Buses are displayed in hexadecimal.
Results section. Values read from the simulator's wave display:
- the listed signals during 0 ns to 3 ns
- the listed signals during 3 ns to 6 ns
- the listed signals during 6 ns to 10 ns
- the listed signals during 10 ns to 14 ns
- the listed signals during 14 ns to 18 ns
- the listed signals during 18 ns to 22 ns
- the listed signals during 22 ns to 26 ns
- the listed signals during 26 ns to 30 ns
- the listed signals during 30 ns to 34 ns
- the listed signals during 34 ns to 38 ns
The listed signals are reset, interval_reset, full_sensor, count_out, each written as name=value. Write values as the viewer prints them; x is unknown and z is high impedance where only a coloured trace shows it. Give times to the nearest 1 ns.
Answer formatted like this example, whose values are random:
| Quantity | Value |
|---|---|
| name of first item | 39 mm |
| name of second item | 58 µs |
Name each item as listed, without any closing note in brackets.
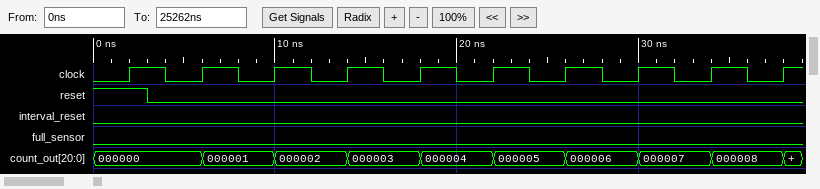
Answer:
| Quantity | Value |
|---|---|
| the listed signals during 0 ns to 3 ns | reset=1, interval_reset=0, full_sensor=0, count_out=000000 |
| the listed signals during 3 ns to 6 ns | reset=0, interval_reset=0, full_sensor=0, count_out=000000 |
| the listed signals during 6 ns to 10 ns | reset=0, interval_reset=0, full_sensor=0, count_out=000001 |
| the listed signals during 10 ns to 14 ns | reset=0, interval_reset=0, full_sensor=0, count_out=000002 |
| the listed signals during 14 ns to 18 ns | reset=0, interval_reset=0, full_sensor=0, count_out=000003 |
| the listed signals during 18 ns to 22 ns | reset=0, interval_reset=0, full_sensor=0, count_out=000004 |
| the listed signals during 22 ns to 26 ns | reset=0, interval_reset=0, full_sensor=0, count_out=000005 |
| the listed signals during 26 ns to 30 ns | reset=0, interval_reset=0, full_sensor=0, count_out=000006 |
| the listed signals during 30 ns to 34 ns | reset=0, interval_reset=0, full_sensor=0, count_out=000007 |
| the listed signals during 34 ns to 38 ns | reset=0, interval_reset=0, full_sensor=0, count_out=000008 |
